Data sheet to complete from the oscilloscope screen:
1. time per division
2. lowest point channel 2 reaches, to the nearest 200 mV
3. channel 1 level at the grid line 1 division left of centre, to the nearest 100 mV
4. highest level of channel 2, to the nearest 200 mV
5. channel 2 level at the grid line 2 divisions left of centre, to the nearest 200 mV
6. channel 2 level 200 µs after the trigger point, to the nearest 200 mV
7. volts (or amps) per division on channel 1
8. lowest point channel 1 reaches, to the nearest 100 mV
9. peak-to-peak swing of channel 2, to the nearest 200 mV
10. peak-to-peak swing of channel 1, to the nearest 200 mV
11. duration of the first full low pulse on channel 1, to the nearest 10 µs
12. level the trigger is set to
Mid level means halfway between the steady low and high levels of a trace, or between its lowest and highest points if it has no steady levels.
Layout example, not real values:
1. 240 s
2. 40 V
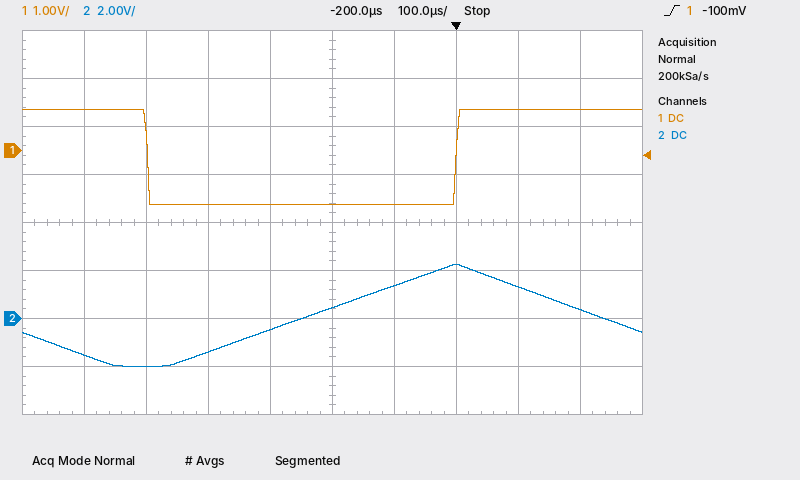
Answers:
1. 100 µs
2. -2.0 V
3. -1.1 V
4. 2.2 V
5. -1.4 V
6. 400 mV
7. 1 V
8. -1.1 V
9. 4.2 V
10. 2.0 V
11. 500 µs
12. -100 mV
